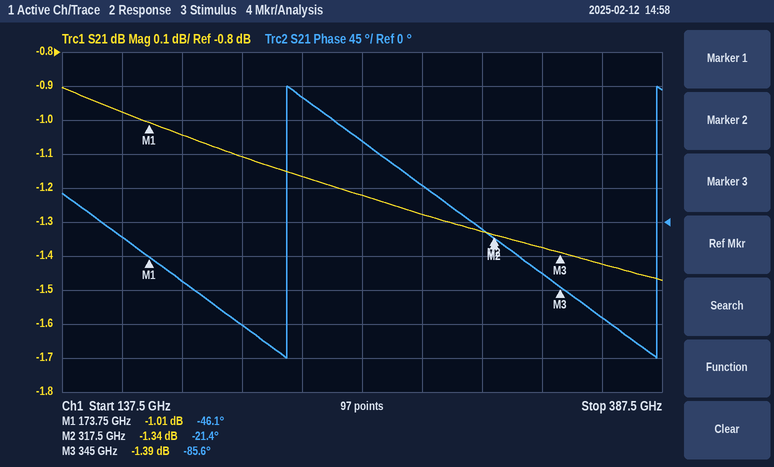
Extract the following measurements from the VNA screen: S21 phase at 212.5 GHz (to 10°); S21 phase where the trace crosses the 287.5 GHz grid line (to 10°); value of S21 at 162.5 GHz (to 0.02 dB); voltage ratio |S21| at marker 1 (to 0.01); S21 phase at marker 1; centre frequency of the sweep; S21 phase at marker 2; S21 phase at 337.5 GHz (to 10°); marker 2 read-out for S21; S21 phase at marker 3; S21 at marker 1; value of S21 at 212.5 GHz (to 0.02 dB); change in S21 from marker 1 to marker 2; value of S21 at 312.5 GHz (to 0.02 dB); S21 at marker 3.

-140°
50°
-0.98 dB
0.89
-46.1°
262.5 GHz
-21.4°
-70°
-1.34 dB
-85.6°
-1.01 dB
-1.10 dB
-0.33 dB
-1.32 dB
-1.39 dB
